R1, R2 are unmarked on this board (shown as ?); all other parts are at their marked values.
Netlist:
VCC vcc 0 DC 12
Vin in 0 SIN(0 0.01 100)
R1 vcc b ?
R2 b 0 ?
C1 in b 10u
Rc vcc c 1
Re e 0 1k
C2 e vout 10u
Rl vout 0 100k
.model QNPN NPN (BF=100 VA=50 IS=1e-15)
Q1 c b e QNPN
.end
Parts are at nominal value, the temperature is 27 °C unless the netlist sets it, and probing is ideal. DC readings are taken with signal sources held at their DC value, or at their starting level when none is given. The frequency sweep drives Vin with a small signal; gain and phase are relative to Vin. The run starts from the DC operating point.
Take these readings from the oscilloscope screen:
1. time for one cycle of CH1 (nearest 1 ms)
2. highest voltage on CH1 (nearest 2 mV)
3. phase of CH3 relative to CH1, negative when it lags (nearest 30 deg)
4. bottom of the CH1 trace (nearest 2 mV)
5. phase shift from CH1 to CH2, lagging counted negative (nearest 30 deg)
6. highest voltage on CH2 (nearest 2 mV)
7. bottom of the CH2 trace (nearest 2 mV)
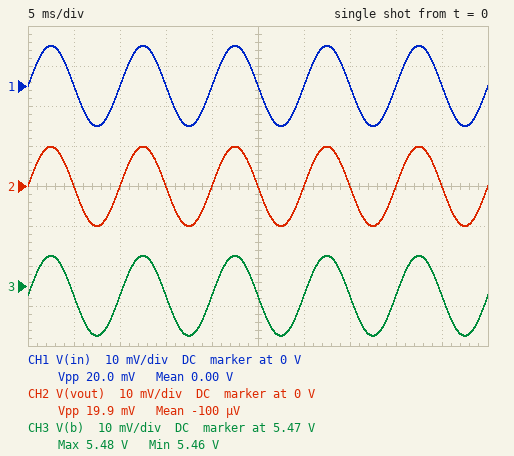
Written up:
10 ms
10 mV
0 deg
-10 mV
0 deg
10 mV
-10 mV
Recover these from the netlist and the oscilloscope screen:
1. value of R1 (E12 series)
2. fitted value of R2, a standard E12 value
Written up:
47 kΩ
56 kΩ
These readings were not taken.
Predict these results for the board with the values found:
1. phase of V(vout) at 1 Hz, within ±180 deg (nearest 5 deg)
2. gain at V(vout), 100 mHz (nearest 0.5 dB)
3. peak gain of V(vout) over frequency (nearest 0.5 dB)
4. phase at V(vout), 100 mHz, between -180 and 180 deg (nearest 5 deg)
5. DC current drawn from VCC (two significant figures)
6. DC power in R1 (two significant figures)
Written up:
45 deg
-23.5 dB
0 dB
140 deg
4.8 mA
910 µW
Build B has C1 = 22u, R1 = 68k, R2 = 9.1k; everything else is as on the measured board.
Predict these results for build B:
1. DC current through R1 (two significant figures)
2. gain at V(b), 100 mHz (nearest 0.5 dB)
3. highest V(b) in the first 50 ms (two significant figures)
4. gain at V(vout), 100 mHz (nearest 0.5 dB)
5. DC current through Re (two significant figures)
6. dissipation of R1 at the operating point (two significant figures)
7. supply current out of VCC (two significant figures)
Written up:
160 µA
-19.5 dB
1.4 V
-25.5 dB
670 µA
1.7 mW
820 µA
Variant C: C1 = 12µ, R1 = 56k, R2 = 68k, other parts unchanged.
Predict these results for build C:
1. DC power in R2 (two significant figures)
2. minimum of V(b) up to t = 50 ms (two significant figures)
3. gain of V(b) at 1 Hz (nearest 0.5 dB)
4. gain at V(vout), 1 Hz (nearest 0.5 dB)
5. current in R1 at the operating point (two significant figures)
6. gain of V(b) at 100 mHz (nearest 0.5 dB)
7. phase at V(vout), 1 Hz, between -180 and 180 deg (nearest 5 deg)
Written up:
420 µW
5.3 V
-1.0 dB
-1.5 dB
120 µA
-15.0 dB
40 deg
